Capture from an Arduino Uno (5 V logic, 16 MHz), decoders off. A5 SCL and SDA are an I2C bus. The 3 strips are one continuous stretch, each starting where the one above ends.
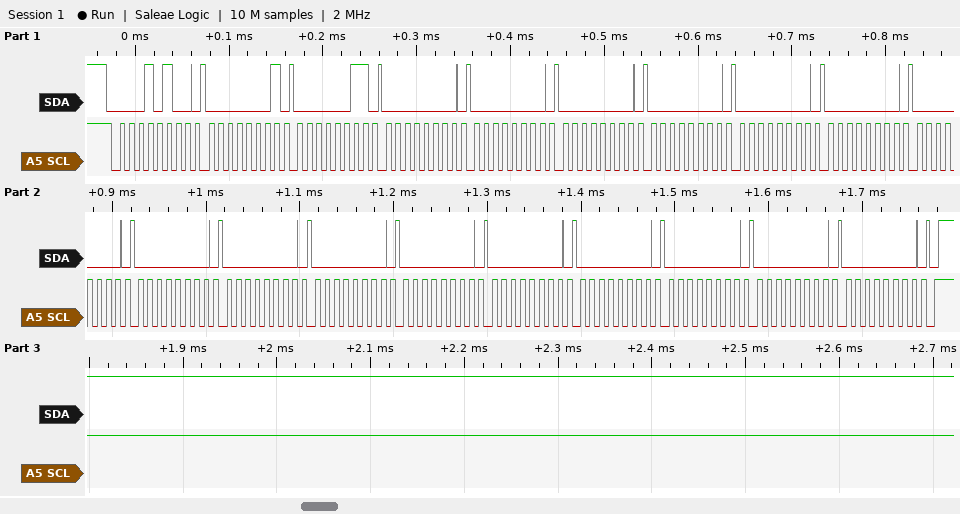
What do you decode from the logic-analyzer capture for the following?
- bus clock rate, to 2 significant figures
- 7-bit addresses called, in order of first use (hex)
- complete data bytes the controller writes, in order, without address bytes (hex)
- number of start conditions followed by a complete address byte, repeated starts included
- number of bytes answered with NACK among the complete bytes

100 kHz
0x0A
01 03 00 00 00 00 00 00 00 00 00 00 00 00 00 00 00 00
1
0
